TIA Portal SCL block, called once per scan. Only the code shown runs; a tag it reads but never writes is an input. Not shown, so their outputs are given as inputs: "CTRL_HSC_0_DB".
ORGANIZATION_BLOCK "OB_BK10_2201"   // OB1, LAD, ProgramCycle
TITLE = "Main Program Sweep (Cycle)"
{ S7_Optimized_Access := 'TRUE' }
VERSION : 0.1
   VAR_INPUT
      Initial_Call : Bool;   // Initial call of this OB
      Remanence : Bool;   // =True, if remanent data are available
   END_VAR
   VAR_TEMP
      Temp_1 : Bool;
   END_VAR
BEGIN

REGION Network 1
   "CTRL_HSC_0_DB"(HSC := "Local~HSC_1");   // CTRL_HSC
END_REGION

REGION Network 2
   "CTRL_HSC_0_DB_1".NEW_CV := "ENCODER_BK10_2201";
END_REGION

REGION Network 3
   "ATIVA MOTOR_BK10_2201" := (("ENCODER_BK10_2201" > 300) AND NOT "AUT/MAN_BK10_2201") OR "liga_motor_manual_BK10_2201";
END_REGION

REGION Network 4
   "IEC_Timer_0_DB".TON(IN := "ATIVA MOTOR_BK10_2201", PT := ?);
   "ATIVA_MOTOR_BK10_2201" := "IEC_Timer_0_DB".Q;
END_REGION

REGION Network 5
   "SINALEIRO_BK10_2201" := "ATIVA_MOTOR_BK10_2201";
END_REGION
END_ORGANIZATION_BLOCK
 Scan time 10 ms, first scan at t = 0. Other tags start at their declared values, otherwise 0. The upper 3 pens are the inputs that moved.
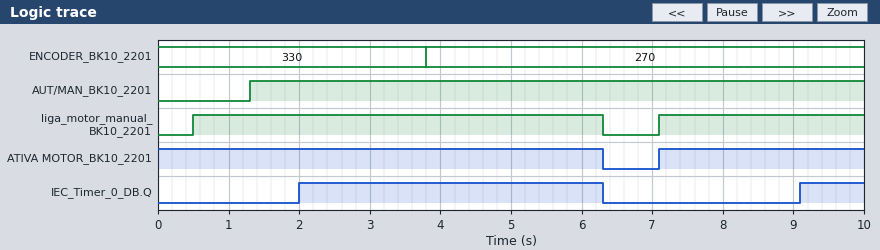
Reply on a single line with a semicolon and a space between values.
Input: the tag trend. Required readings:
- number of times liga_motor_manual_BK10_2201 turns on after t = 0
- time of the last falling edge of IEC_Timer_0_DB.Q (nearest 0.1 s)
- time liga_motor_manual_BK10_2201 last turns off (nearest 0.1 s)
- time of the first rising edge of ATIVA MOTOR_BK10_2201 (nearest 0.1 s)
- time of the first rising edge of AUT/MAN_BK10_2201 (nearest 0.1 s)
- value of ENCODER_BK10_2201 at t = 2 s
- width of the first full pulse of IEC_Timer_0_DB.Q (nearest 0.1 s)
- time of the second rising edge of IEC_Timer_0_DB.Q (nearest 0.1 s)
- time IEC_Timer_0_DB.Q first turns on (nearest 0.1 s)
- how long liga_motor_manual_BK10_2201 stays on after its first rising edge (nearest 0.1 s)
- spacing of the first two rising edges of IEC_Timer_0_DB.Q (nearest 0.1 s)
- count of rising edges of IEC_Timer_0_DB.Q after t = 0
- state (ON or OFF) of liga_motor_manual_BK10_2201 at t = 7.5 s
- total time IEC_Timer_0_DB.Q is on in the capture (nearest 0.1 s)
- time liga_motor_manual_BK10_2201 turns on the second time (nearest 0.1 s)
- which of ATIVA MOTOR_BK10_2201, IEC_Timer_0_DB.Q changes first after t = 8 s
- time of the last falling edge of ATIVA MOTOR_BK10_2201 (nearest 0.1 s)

2; 6.3 s; 6.3 s; 7.1 s; 1.3 s; 330; 4.3 s; 9.1 s; 2.0 s; 5.8 s; 7.1 s; 2; ON; 5.2 s; 7.1 s; IEC_Timer_0_DB.Q; 6.3 s
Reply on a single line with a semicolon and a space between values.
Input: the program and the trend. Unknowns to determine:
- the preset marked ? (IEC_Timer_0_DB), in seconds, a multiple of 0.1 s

2.0 s
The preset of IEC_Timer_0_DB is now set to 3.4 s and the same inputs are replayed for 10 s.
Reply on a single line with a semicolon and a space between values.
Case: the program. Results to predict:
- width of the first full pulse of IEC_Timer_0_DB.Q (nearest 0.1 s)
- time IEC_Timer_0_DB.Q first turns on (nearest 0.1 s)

2.9 s; 3.4 s
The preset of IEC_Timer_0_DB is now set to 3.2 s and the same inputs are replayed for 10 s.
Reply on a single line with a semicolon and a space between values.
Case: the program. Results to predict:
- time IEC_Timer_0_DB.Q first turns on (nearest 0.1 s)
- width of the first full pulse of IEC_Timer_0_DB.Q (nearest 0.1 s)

3.2 s; 3.1 s
